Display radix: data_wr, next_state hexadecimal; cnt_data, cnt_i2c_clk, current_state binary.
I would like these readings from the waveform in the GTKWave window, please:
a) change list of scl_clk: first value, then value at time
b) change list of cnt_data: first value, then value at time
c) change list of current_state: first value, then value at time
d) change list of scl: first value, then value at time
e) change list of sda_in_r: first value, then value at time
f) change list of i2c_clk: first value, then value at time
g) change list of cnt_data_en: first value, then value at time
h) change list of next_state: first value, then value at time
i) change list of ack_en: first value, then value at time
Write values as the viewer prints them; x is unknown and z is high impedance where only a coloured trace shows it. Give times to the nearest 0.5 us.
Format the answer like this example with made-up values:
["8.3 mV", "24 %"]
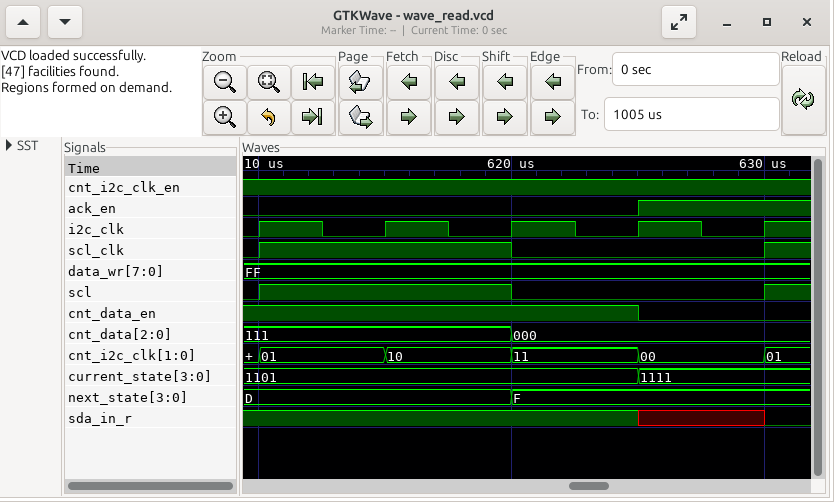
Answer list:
["0, 1 at 610 us, 0 at 620 us, 1 at 630 us", "111, 000 at 620 us", "1101, 1111 at 625 us", "0, 1 at 610 us, 0 at 620 us, 1 at 630 us", "1, x at 625 us, 0 at 630 us", "0, 1 at 610 us, 0 at 612.5 us, 1 at 615 us, 0 at 617.5 us, 1 at 620 us, 0 at 622.5 us, 1 at 625 us, 0 at 627.5 us, 1 at 630 us", "1, 0 at 625 us", "D, F at 620 us", "0, 1 at 625 us"]
